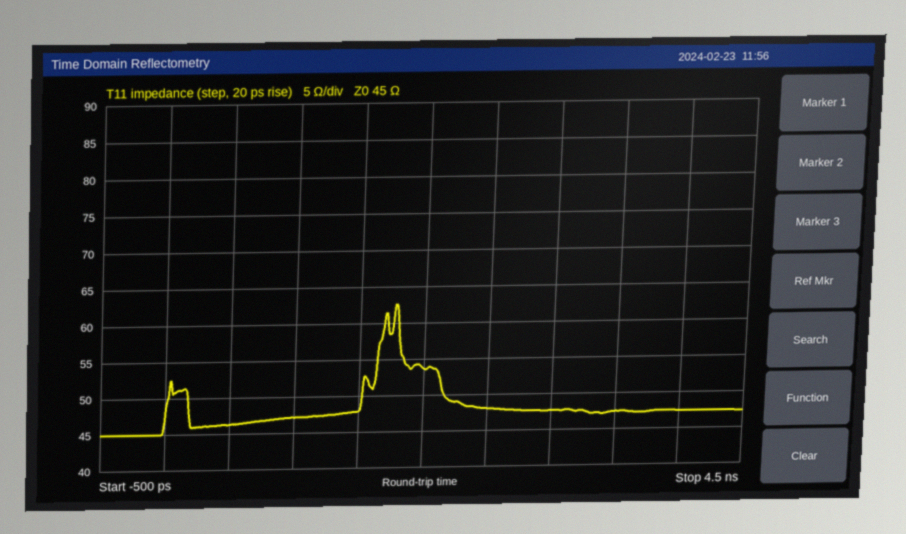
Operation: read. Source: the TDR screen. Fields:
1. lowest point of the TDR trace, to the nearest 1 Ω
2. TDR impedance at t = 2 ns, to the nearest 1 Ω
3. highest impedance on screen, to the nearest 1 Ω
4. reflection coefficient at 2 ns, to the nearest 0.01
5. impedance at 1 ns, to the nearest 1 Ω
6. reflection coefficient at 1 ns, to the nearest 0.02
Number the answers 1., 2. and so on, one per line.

1. 45 Ω
2. 54 Ω
3. 63 Ω
4. +0.09
5. 47 Ω
6. +0.02
